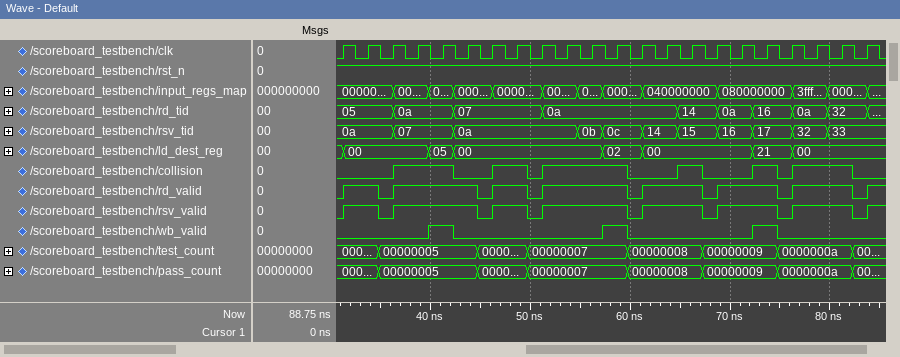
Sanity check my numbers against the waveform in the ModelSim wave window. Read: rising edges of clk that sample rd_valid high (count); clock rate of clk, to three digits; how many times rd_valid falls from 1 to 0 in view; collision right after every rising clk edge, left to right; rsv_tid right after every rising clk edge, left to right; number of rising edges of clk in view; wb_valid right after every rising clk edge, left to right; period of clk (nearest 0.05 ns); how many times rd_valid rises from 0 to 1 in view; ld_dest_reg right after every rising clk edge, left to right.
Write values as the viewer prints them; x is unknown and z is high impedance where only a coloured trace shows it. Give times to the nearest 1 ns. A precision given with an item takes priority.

14
400 MHz
7
0 0 1 1 1 0 1 1 1 1 1 1 0 0 1 0 0 1 1 1 1 0
0a, 0a, 07, 07, 07, 0a, 0a, 0a, 0a, 0a, 0b, 0c, 14, 14, 15, 16, 16, 17, 32, 32, 33, 33
22
0 0 0 0 1 0 0 0 0 0 0 1 0 0 0 0 0 1 0 0 0 0
2.5 ns
8
00, 00, 00, 00, 05, 00, 00, 00, 00, 00, 00, 02, 00, 00, 00, 00, 00, 21, 00, 00, 00, 00
